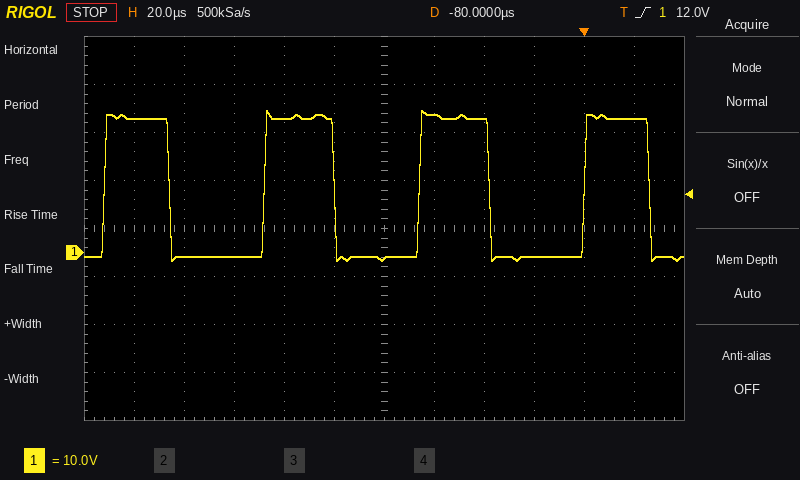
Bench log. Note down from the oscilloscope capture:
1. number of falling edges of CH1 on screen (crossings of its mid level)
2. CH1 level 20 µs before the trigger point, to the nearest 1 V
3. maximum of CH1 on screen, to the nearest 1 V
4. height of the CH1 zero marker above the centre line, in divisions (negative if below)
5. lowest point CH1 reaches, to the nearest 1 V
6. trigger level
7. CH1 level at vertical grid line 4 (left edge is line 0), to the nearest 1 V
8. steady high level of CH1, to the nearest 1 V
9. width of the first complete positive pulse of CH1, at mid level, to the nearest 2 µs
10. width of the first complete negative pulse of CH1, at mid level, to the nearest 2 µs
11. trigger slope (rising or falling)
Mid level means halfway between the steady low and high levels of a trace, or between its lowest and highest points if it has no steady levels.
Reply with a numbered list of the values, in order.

1. 4
2. -1 V
3. 30 V
4. -0.5 div
5. -2 V
6. 12.0 V
7. 28 V
8. 28 V
9. 26 µs
10. 38 µs
11. rising
